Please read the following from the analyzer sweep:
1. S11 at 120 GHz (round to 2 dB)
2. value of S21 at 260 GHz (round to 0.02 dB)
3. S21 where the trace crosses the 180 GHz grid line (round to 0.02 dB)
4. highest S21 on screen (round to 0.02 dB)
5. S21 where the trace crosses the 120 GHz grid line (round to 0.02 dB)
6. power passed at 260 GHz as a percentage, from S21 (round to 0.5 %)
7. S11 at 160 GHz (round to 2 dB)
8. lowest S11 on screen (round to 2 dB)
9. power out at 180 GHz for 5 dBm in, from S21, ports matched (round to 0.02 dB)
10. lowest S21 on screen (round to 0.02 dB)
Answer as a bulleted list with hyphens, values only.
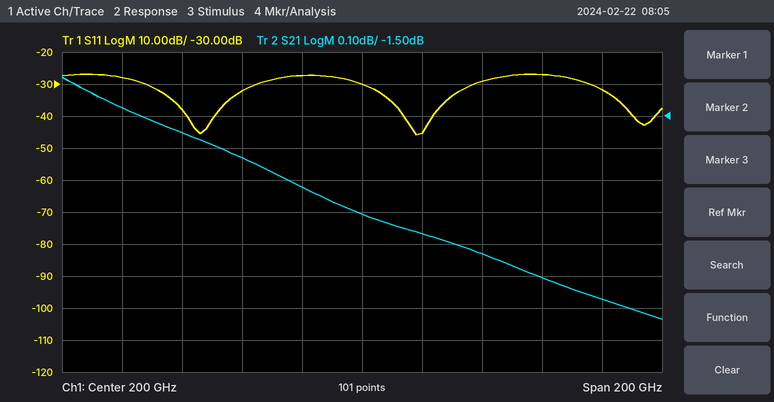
- -28 dB
- -2.00 dB
- -1.72 dB
- -1.38 dB
- -1.48 dB
- 63.0 %
- -32 dB
- -46 dB
- 3.28 dBm
- -2.14 dB
